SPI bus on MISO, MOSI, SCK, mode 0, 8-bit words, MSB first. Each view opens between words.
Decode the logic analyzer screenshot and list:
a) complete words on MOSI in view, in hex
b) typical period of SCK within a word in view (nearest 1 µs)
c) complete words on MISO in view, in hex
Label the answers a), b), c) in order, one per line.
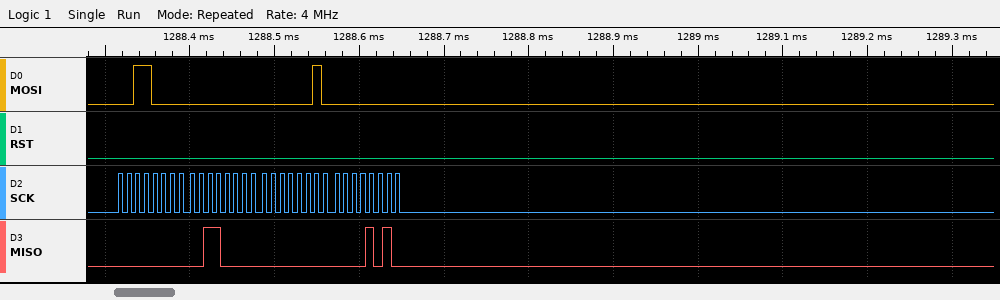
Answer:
a) 30, 00, 02, 00
b) 10 µs
c) 00, 30, 00, 0A
